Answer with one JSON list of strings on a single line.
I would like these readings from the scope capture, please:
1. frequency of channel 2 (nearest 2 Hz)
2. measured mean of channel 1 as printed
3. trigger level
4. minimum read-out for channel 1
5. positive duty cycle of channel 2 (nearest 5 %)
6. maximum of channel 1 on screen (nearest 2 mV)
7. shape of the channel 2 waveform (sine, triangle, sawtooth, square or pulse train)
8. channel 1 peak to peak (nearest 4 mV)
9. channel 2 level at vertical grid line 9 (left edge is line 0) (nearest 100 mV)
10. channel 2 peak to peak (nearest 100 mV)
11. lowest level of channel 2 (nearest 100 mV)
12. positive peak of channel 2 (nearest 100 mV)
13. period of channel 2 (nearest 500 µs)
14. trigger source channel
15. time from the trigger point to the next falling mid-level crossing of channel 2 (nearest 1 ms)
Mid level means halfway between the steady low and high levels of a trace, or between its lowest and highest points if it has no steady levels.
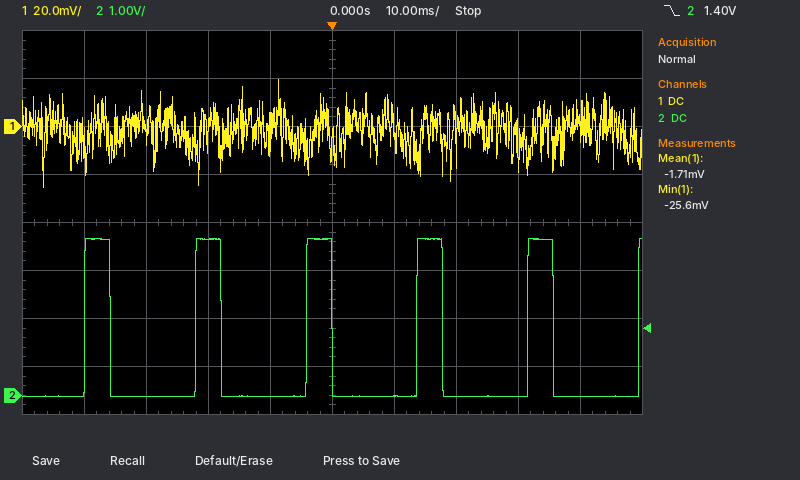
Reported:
["56 Hz", "-1.71 mV", "1.40 V", "-25.6 mV", "25 %", "20 mV", "pulse train", "44 mV", "0.0 V", "3.3 V", "0.0 V", "3.3 V", "18.0 ms", "channel 2", "18 ms"]
